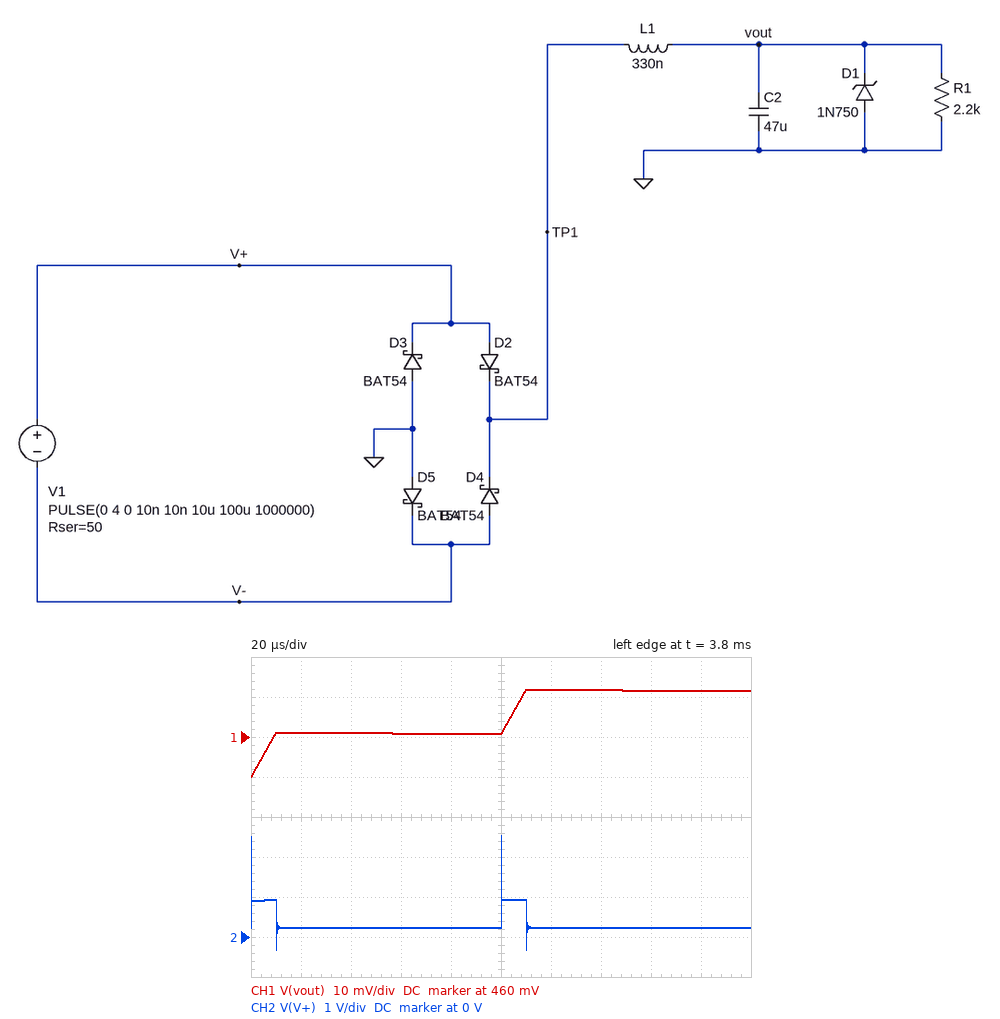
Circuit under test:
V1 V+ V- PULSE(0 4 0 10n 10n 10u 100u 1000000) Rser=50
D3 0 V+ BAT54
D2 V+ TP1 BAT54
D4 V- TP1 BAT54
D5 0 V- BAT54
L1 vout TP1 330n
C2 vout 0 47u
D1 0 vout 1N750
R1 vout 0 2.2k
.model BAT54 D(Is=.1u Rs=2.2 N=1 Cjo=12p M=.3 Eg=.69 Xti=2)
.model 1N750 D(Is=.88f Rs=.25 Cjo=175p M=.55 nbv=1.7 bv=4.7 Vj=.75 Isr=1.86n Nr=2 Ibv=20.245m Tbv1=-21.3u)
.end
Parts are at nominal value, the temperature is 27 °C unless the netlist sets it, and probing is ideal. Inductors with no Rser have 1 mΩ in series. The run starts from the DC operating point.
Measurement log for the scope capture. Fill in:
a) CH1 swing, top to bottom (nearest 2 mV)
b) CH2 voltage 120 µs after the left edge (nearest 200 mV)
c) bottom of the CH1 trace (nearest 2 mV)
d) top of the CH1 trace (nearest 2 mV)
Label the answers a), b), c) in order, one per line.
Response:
a) 22 mV
b) 200 mV
c) 450 mV
d) 472 mV
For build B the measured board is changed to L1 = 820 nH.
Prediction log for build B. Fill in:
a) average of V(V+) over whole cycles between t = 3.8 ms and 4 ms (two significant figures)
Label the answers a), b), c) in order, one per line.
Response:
a) 300 mV
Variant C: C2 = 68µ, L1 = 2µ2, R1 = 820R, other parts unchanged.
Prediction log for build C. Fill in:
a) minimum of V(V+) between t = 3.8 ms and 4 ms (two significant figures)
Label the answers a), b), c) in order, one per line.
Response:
a) -380 mV
